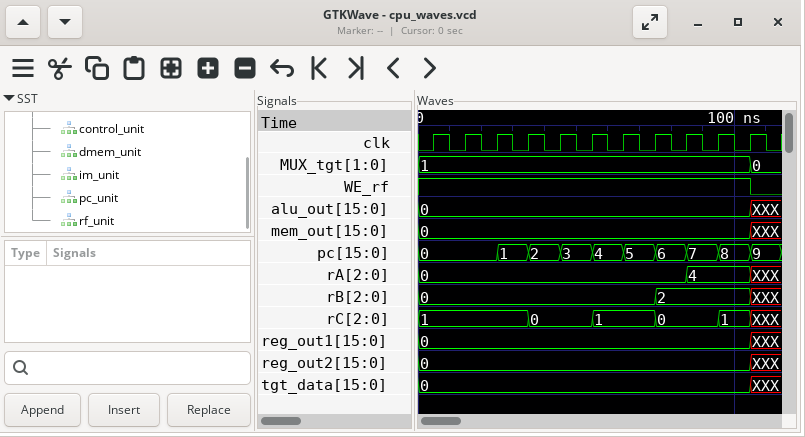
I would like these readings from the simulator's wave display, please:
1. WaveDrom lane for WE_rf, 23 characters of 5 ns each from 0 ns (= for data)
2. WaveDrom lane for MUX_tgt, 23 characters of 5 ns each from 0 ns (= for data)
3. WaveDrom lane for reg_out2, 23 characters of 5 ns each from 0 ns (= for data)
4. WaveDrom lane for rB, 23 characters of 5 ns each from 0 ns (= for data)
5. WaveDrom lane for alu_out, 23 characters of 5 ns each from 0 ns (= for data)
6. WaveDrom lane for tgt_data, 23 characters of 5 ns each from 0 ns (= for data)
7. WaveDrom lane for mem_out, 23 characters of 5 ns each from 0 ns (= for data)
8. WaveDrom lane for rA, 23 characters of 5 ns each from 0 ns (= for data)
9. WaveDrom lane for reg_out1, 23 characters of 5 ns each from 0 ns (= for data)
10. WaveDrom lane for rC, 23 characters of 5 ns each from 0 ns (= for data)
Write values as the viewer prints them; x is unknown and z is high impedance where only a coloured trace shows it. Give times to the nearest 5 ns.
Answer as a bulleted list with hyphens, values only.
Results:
- {name: 'WE_rf', wave: '1....................0.'}
- {name: 'MUX_tgt', wave: '=....................=.', data: '1 0'}
- {name: 'reg_out2', wave: '=....................x.', data: '0'}
- {name: 'rB', wave: '=..............=.....x.', data: '0 2'}
- {name: 'alu_out', wave: '=....................x.', data: '0'}
- {name: 'tgt_data', wave: '=....................x.', data: '0'}
- {name: 'mem_out', wave: '=....................x.', data: '0'}
- {name: 'rA', wave: '=................=...x.', data: '0 4'}
- {name: 'reg_out1', wave: '=....................x.', data: '0'}
- {name: 'rC', wave: '=......=...=...=...=.x.', data: '1 0 1 0 1'}
